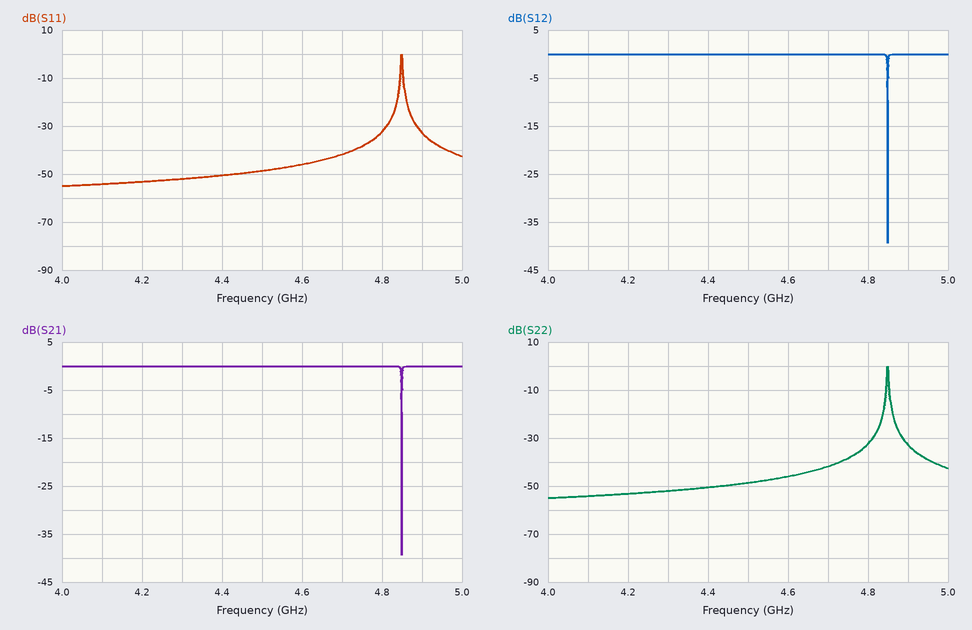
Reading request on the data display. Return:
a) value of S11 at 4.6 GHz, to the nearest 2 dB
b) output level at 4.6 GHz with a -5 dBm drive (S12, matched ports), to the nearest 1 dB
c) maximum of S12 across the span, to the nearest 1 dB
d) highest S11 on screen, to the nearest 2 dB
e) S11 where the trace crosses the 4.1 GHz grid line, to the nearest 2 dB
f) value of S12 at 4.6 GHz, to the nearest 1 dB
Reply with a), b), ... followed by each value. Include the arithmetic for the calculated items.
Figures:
a) -46 dB
b) -5 dBm + (0 dB) = -5 dBm
c) 0 dB
d) 0 dB
e) -54 dB
f) 0 dB
